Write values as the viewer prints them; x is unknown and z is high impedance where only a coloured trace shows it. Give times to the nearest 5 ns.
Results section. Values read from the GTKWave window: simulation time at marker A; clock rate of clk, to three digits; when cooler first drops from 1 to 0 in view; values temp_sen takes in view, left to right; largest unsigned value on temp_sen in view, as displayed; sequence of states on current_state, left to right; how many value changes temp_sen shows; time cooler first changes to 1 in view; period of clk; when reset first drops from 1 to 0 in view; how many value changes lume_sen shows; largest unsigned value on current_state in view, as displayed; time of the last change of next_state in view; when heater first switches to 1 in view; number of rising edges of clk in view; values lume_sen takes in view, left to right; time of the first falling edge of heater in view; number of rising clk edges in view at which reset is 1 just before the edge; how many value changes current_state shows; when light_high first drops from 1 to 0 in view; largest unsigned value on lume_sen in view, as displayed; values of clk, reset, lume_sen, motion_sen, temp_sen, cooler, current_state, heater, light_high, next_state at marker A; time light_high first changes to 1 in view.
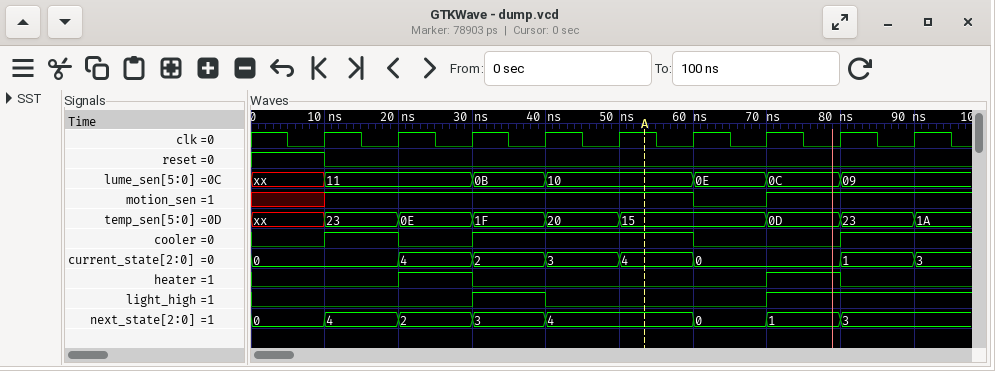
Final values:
55 ns
100 MHz
20 ns
xx, 23, 0E, 1F, 20, 15, 0D, 23, 1A
23
0, 4, 2, 3, 4, 0, 1, 3
8
10 ns
10 ns
10 ns
6
4
80 ns
20 ns
9
xx, 11, 0B, 10, 0E, 0C, 09
30 ns
1
7
40 ns
11
clk=1, reset=0, lume_sen=10, motion_sen=1, temp_sen=15, cooler=1, current_state=4, heater=0, light_high=0, next_state=4
30 ns
